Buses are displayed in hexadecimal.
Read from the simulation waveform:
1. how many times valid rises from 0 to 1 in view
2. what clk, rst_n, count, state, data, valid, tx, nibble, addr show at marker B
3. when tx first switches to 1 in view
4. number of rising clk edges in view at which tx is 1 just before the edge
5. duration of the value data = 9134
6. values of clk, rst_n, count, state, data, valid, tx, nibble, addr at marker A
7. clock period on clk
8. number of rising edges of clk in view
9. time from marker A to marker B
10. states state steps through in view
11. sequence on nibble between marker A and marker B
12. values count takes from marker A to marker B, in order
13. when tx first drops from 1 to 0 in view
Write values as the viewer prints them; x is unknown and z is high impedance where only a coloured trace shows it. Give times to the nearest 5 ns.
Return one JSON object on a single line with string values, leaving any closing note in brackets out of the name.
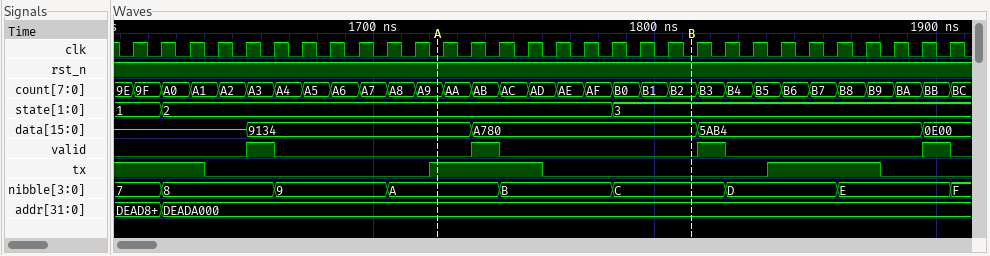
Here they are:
{"how many times valid rises from 0 to 1 in view": "4", "what clk, rst_n, count, state, data, valid, tx, nibble, addr show at marker B": "clk=0, rst_n=1, count=B2, state=3, data=A780, valid=0, tx=0, nibble=C, addr=DEADA000", "when tx first switches to 1 in view": "1720 ns", "number of rising clk edges in view at which tx is 1 just before the edge": "11", "duration of the value data = 9134": "80 ns", "values of clk, rst_n, count, state, data, valid, tx, nibble, addr at marker A": "clk=0, rst_n=1, count=A9, state=2, data=9134, valid=0, tx=1, nibble=A, addr=DEADA000", "clock period on clk": "10 ns", "number of rising edges of clk in view": "30", "time from marker A to marker B": "90 ns", "states state steps through in view": "1, 2, 3", "sequence on nibble between marker A and marker B": "A, B, C", "values count takes from marker A to marker B, in order": "A9, AA, AB, AC, AD, AE, AF, B0, B1, B2", "when tx first drops from 1 to 0 in view": "1640 ns"}
